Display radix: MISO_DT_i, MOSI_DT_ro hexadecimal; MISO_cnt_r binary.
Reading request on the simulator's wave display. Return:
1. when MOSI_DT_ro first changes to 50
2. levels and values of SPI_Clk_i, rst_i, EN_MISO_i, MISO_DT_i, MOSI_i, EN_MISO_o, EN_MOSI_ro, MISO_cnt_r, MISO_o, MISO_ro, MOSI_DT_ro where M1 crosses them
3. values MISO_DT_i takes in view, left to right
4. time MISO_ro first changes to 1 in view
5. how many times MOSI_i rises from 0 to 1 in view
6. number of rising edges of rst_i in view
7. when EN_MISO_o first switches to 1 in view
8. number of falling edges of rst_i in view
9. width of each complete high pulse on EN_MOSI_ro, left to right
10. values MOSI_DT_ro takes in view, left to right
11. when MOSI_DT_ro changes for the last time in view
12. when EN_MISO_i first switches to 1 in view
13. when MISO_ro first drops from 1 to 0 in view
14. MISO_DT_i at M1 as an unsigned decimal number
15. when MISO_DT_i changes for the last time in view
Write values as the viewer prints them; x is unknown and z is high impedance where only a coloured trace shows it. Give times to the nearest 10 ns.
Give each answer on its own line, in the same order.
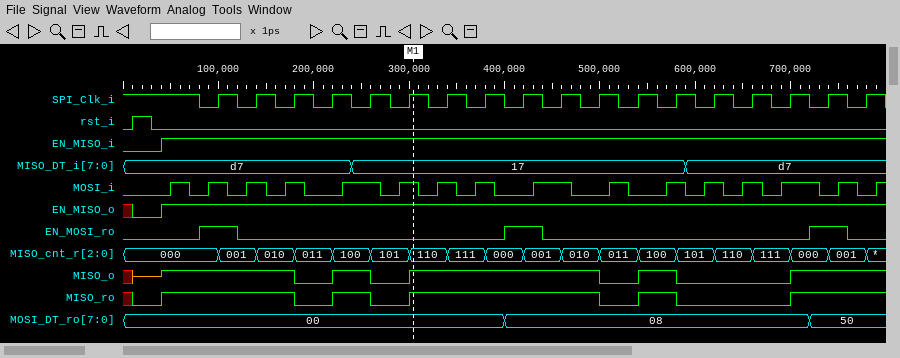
720 ns
SPI_Clk_i=1, rst_i=0, EN_MISO_i=1, MISO_DT_i=17, MOSI_i=1, EN_MISO_o=1, EN_MOSI_ro=0, MISO_cnt_r=110, MISO_o=1, MISO_ro=1, MOSI_DT_ro=00
d7, 17, d7
40 ns
16
1
40 ns
1
40 ns, 40 ns, 40 ns
00, 08, 50
720 ns
40 ns
180 ns
23
590 ns
